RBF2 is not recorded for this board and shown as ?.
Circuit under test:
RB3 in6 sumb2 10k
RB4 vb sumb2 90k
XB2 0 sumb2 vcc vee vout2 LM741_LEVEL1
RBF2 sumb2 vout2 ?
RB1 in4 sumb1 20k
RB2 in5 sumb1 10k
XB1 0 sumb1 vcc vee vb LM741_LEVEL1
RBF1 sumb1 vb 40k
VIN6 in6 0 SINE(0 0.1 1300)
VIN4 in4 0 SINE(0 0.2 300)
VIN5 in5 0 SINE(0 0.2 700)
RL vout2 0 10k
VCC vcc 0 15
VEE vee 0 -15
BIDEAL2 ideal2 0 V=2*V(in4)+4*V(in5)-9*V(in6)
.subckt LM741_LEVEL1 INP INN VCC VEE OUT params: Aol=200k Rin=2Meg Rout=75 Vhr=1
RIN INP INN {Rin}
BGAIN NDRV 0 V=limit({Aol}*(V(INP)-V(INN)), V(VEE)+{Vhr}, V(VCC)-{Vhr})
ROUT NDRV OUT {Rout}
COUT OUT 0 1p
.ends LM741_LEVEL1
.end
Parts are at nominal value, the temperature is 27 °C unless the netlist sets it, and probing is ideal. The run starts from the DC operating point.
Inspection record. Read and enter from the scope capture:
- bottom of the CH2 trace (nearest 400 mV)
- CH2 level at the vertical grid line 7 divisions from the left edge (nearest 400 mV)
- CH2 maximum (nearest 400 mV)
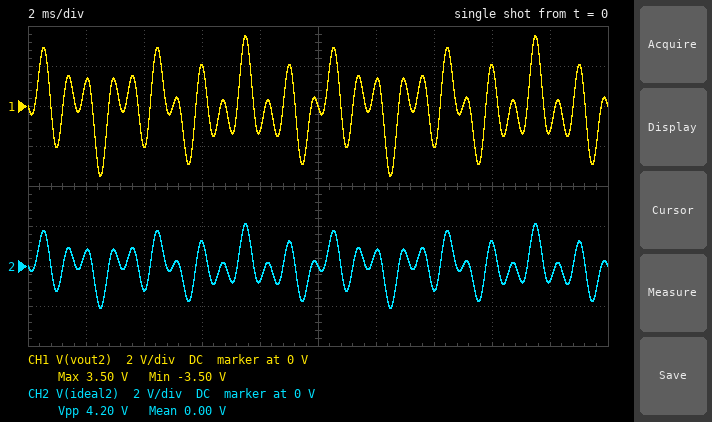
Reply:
-2.0 V
-1.2 V
2.0 V
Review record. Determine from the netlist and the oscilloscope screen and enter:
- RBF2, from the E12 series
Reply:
150 kΩ
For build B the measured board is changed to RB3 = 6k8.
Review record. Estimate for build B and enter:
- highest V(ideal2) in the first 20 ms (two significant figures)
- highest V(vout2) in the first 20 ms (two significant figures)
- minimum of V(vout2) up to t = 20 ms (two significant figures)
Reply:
2.1 V
4.2 V
-4.2 V
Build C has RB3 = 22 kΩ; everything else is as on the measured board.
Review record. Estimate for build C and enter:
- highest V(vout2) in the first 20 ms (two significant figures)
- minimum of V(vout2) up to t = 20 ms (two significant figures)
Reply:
2.7 V
-2.7 V
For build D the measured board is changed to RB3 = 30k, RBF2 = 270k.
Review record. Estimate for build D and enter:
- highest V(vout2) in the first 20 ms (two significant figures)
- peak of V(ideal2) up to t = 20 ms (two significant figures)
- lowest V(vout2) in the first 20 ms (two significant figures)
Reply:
4.5 V
2.1 V
-4.5 V
